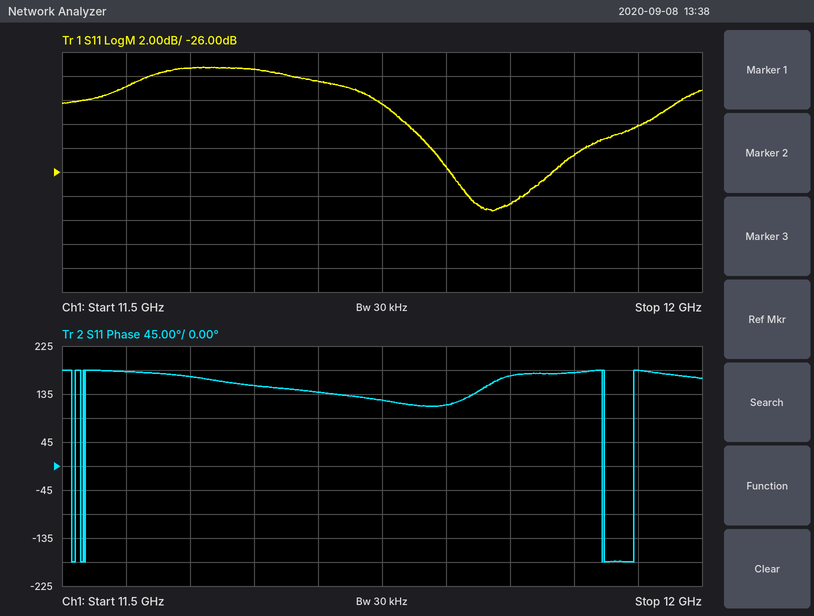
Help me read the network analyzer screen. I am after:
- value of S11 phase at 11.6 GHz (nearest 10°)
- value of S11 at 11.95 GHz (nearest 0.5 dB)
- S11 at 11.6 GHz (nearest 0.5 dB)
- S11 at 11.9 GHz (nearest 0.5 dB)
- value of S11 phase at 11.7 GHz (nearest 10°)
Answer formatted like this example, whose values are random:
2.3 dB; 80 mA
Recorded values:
170°; -22.0 dB; -17.5 dB; -24.5 dB; 140°
